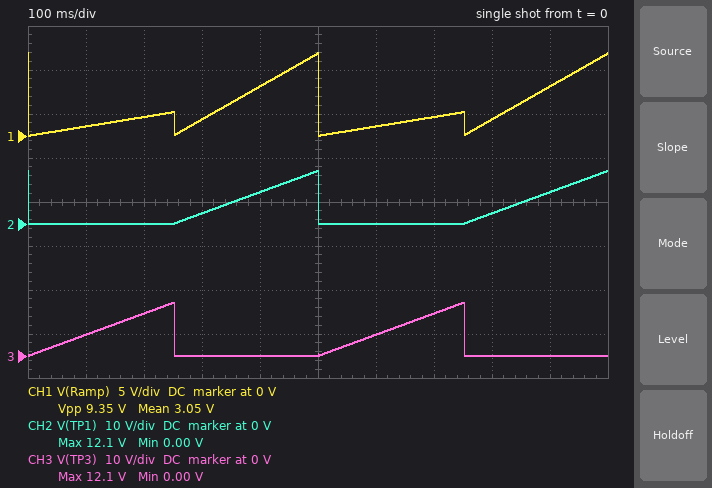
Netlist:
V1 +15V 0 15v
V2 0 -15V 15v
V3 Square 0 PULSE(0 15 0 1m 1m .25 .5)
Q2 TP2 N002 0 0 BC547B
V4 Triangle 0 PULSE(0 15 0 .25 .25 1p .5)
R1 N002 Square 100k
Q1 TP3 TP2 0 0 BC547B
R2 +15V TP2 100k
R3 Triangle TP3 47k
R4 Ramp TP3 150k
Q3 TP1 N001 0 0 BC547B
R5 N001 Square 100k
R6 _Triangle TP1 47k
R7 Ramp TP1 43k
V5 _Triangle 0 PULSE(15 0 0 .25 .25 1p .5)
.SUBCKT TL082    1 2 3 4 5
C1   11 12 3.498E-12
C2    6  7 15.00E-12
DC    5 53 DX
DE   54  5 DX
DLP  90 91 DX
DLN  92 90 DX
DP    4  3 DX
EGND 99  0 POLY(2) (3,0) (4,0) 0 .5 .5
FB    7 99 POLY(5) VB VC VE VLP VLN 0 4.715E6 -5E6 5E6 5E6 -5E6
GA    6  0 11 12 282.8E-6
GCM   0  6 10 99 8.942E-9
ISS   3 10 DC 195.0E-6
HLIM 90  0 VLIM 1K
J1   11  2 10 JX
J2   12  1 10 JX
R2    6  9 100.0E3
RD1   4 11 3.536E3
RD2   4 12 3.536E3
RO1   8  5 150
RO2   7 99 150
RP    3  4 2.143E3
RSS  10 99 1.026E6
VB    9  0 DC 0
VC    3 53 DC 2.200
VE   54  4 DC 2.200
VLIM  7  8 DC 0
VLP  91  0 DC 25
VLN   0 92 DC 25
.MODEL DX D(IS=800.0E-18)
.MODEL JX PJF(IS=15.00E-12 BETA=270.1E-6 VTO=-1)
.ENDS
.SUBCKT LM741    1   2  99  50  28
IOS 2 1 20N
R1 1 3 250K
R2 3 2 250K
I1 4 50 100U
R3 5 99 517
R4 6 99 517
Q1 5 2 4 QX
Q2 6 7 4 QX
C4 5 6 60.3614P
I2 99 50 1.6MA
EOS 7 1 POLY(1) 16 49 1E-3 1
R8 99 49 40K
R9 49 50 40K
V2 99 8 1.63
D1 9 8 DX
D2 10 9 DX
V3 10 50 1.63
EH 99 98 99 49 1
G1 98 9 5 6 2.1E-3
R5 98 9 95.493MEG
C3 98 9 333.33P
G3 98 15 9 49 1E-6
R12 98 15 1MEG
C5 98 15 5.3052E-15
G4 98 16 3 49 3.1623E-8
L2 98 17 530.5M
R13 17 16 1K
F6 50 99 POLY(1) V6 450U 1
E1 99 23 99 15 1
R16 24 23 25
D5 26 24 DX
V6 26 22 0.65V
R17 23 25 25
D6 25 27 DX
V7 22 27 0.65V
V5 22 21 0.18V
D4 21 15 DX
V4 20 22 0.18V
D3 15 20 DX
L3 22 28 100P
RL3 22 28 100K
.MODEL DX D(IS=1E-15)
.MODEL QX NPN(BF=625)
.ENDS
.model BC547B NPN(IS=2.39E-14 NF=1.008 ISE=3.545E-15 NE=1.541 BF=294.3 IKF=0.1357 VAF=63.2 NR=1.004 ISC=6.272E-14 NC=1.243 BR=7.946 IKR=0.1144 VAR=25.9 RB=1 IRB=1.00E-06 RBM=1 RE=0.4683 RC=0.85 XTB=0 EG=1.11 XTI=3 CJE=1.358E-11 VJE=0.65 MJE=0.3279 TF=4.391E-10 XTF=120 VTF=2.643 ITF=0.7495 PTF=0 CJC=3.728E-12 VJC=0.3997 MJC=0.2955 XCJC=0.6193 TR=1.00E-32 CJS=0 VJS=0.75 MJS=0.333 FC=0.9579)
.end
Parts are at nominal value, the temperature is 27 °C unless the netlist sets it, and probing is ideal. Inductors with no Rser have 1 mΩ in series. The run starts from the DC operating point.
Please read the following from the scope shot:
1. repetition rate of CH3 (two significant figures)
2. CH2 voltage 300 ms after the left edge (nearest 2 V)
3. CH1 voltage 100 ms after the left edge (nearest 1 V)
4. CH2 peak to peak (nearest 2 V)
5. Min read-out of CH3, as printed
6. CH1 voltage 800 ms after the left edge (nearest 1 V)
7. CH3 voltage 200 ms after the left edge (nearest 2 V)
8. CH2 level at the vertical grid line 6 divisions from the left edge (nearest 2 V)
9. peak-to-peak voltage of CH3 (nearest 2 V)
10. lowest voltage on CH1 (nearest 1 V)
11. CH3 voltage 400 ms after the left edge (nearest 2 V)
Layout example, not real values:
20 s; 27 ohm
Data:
2.0 Hz; 2 V; 1 V; 12 V; 0.00 V; 2 V; 10 V; 0 V; 12 V; 0 V; 0 V
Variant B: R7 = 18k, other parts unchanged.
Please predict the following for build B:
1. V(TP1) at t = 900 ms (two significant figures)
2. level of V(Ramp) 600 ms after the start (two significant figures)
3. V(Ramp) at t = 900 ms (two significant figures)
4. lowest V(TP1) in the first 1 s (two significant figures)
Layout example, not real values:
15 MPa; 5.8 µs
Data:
7.0 V; 510 mV; 6.3 V; 8.2 mV
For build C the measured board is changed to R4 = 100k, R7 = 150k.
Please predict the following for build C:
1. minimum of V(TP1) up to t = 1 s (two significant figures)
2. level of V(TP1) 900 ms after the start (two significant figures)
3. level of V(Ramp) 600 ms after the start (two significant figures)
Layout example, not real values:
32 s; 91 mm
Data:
7.7 mV; 7.6 V; 3.0 V
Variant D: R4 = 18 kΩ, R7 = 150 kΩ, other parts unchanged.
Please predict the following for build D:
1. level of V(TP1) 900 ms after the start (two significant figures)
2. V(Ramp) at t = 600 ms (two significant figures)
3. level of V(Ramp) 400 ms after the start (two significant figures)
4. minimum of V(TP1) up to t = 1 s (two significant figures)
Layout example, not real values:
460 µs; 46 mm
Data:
7.0 V; 4.2 V; 760 mV; 8.2 mV
